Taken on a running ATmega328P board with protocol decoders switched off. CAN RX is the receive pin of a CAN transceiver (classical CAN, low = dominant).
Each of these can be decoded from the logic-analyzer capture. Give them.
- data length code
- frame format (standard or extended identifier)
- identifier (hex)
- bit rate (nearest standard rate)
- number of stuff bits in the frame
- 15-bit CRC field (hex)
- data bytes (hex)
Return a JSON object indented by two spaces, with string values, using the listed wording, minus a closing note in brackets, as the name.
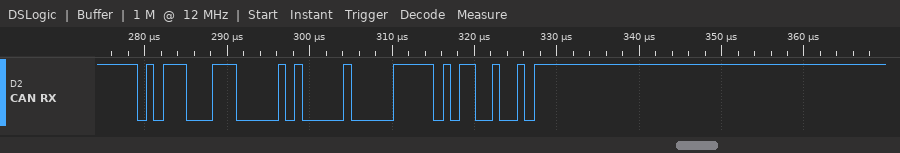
{
  "data length code": "1",
  "frame format": "standard",
  "identifier": "0x5C7",
  "bit rate": "1000 kbit/s",
  "number of stuff bits in the frame": "4",
  "15-bit CRC field": "0x1F64",
  "data bytes": "00"
}
